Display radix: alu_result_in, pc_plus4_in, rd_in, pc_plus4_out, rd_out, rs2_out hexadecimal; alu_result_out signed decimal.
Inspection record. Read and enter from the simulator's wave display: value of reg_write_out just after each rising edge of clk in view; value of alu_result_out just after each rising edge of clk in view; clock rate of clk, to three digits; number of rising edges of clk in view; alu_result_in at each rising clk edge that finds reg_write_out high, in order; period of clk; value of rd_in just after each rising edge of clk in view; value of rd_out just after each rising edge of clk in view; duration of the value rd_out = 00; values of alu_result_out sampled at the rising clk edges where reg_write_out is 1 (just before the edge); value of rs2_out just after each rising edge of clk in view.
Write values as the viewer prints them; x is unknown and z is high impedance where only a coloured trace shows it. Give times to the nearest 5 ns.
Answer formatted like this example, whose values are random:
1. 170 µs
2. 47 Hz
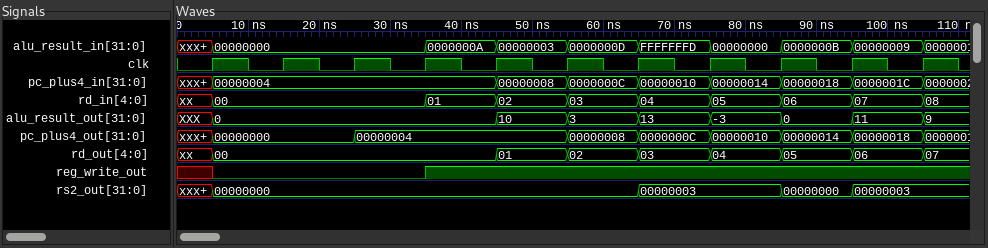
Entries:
1. 0 0 0 1 1 1 1 1 1 1 1
2. 0, 0, 0, 0, 10, 3, 13, -3, 0, 11, 9
3. 100 MHz
4. 11
5. 0000000A, 00000003, 0000000D, FFFFFFFD, 00000000, 0000000B, 00000009
6. 10 ns
7. 00, 00, 00, 01, 02, 03, 04, 05, 06, 07, 08
8. 00, 00, 00, 00, 01, 02, 03, 04, 05, 06, 07
9. 40 ns
10. 0, 10, 3, 13, -3, 0, 11
11. 00000000, 00000000, 00000000, 00000000, 00000000, 00000000, 00000003, 00000003, 00000000, 00000003, 00000003
